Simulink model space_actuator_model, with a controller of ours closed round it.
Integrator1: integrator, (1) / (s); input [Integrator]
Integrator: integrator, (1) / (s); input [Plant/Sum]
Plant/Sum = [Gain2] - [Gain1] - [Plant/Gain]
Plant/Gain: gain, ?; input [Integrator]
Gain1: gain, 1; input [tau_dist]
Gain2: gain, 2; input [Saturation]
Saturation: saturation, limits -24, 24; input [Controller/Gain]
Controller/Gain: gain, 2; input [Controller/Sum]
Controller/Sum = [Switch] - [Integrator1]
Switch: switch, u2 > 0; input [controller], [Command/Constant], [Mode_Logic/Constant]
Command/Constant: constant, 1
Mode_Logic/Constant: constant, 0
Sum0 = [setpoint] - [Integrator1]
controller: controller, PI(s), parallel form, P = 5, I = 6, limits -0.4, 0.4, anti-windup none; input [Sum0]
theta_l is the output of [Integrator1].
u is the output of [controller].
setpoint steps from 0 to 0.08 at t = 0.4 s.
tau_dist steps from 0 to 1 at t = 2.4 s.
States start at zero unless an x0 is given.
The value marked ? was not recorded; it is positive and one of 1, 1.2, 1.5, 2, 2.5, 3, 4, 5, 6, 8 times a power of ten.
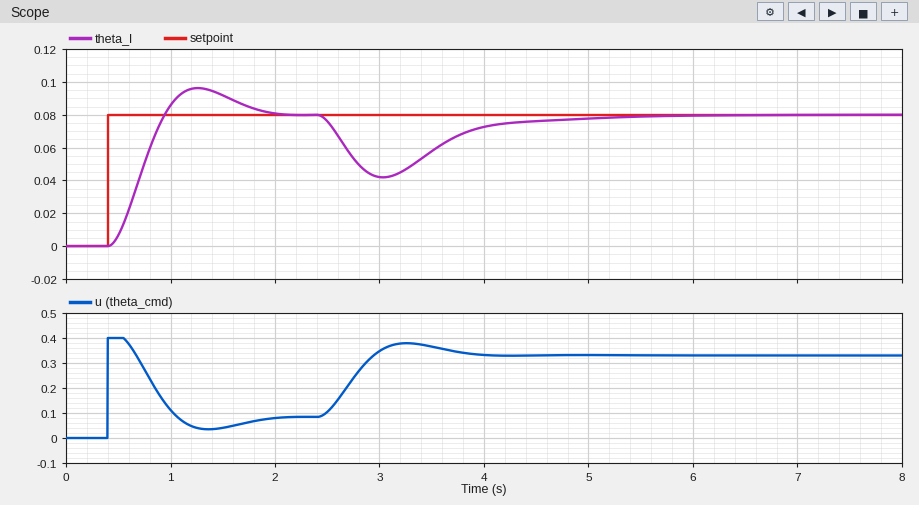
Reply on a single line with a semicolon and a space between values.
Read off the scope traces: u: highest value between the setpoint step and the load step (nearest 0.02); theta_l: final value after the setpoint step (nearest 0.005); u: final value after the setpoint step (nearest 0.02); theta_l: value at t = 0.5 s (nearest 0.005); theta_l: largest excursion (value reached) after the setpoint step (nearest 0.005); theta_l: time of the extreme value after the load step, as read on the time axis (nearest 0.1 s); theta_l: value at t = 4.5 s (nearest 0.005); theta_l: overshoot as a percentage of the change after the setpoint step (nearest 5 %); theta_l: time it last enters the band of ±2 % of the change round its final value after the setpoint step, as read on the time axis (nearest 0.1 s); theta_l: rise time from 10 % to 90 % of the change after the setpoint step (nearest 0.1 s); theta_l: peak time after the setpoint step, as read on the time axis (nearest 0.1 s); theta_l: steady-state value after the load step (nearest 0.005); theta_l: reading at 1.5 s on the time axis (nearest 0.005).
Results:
0.40; 0.080; 0.08; 0.005; 0.095; 3.0 s; 0.075; 20 %; 1.9 s; 0.4 s; 1.3 s; 0.080; 0.090
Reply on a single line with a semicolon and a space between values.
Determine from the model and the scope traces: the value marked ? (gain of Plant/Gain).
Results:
6
